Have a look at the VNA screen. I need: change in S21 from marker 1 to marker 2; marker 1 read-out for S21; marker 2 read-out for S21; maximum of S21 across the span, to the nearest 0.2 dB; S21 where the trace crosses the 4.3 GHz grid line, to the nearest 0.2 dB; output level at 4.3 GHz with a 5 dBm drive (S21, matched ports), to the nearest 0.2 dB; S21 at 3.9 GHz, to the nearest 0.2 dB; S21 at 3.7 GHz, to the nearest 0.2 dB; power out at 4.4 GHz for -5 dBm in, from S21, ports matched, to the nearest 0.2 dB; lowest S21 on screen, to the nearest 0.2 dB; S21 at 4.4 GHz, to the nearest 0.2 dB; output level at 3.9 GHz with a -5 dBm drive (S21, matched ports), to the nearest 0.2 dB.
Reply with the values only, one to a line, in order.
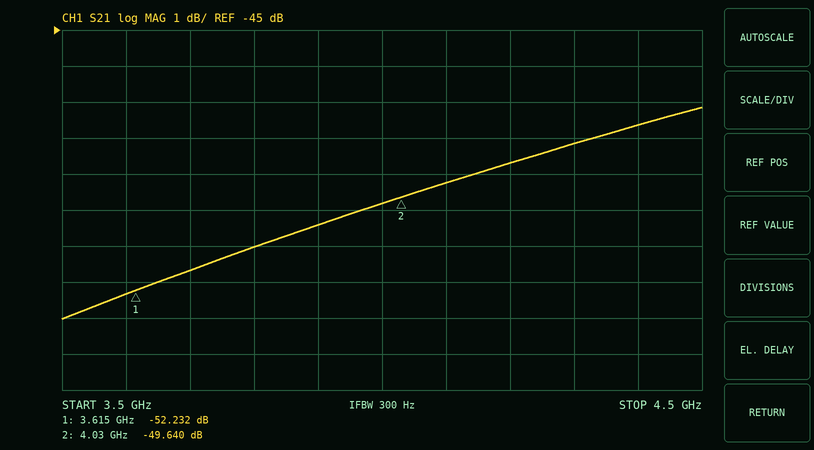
2.592 dB
-52.232 dB
-49.640 dB
-47.2 dB
-48.2 dB
-43.2 dBm
-50.4 dB
-51.6 dB
-52.6 dBm
-53.0 dB
-47.6 dB
-55.4 dBm
